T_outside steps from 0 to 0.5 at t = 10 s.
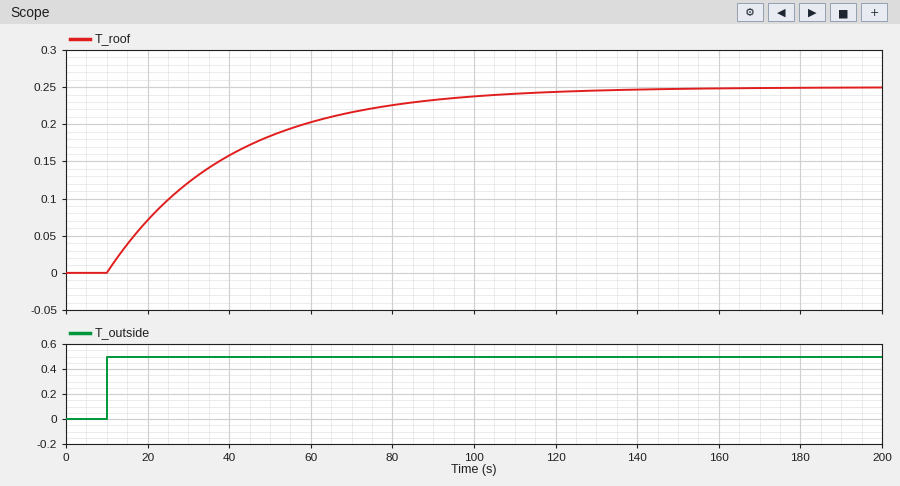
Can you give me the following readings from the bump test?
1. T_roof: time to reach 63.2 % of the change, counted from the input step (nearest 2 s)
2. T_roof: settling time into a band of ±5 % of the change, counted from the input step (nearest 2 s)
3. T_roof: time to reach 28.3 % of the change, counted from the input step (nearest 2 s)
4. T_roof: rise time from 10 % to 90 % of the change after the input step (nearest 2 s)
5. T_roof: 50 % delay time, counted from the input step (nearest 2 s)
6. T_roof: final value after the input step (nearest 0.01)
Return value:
30 s
90 s
10 s
66 s
20 s
0.25
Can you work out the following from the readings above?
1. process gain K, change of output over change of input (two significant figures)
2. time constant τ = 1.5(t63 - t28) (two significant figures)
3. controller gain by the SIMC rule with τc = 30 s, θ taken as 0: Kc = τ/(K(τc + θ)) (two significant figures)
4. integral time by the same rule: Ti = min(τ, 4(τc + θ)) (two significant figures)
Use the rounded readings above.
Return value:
0.50
30 s
2.0
30 s
